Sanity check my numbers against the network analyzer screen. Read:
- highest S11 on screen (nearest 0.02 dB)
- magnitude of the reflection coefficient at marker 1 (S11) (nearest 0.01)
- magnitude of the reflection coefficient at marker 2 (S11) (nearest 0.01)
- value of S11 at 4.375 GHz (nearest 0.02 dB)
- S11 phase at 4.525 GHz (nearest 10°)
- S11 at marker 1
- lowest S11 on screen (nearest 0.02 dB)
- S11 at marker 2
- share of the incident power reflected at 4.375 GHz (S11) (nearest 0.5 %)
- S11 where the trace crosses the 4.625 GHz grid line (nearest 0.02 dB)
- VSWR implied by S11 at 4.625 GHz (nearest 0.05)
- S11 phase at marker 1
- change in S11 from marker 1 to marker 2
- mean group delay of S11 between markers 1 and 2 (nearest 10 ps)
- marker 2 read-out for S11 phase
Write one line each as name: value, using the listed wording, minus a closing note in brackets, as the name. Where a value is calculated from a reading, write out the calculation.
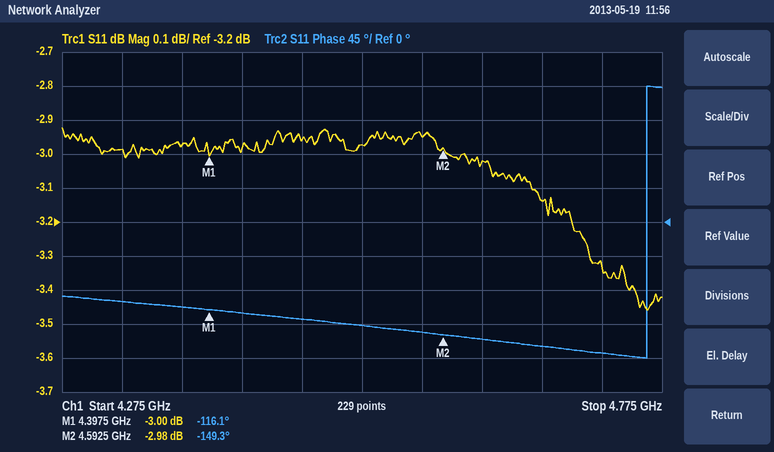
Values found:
highest S11 on screen: -2.92 dB
magnitude of the reflection coefficient at marker 1 (S11): 10^(-3/20) ≈ 0.71
magnitude of the reflection coefficient at marker 2 (S11): 10^(-2.98/20) ≈ 0.71
value of S11 at 4.375 GHz: -2.98 dB
S11 phase at 4.525 GHz: -140°
S11 at marker 1: -3.00 dB
lowest S11 on screen: -3.46 dB
S11 at marker 2: -2.98 dB
share of the incident power reflected at 4.375 GHz (S11): 10^(-2.98/10) ≈ 50.4 %, so 50.5 % to the nearest 0.5 %
S11 where the trace crosses the 4.625 GHz grid line: -3.02 dB
VSWR implied by S11 at 4.625 GHz: |Γ| = 10^(-3.02/20) = 0.7063; VSWR = (1 + 0.7063)/(1 − 0.7063) ≈ 5.81, so 5.80 to the nearest 0.05
S11 phase at marker 1: -116.1°
change in S11 from marker 1 to marker 2: -2.98 − (-3) = 0.02 dB
mean group delay of S11 between markers 1 and 2: −(-149.3° − (-116.1°))/(360° × 195 MHz) ≈ 473 ps, so 470 ps to the nearest 10 ps
marker 2 read-out for S11 phase: -149.3°
